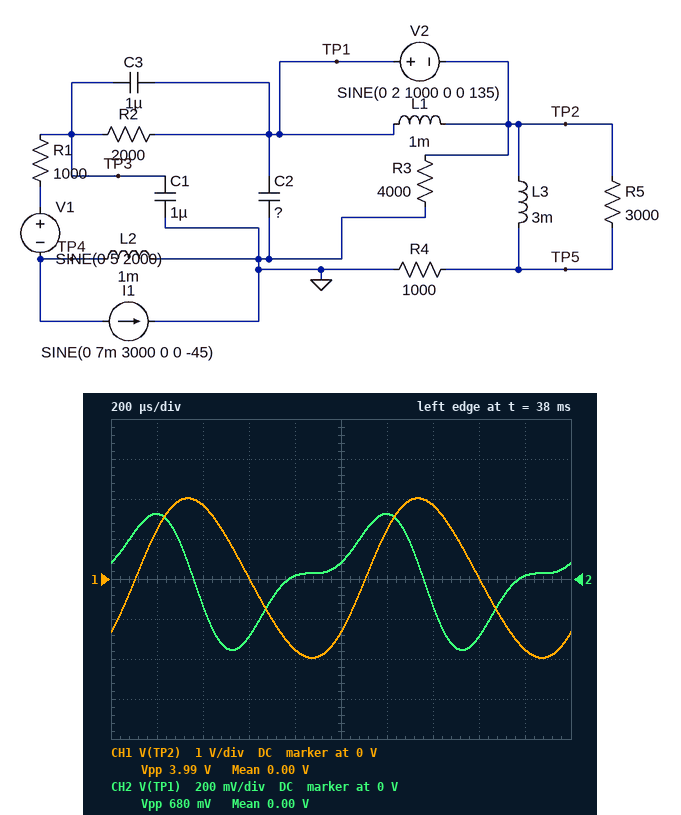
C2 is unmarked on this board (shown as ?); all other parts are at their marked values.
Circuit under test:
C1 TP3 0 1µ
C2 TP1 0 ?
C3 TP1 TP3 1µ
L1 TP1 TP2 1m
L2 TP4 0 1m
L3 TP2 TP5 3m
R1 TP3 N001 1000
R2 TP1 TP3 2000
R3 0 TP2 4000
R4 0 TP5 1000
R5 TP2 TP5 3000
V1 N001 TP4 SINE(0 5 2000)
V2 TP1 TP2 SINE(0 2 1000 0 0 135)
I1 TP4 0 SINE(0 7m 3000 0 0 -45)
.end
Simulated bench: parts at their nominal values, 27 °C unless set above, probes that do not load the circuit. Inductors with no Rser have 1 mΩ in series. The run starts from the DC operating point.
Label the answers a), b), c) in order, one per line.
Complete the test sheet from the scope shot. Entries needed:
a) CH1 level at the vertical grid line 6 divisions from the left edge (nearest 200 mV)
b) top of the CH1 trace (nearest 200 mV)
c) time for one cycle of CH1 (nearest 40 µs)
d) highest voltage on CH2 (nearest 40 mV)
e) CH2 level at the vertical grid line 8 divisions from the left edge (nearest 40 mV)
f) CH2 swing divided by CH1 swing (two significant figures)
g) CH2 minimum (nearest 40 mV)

a) 1.2 V
b) 2.0 V
c) 1.00 ms
d) 320 mV
e) -280 mV
f) 0.17
g) -360 mV
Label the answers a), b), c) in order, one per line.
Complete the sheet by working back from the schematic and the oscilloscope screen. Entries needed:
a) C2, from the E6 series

a) 1 µF
